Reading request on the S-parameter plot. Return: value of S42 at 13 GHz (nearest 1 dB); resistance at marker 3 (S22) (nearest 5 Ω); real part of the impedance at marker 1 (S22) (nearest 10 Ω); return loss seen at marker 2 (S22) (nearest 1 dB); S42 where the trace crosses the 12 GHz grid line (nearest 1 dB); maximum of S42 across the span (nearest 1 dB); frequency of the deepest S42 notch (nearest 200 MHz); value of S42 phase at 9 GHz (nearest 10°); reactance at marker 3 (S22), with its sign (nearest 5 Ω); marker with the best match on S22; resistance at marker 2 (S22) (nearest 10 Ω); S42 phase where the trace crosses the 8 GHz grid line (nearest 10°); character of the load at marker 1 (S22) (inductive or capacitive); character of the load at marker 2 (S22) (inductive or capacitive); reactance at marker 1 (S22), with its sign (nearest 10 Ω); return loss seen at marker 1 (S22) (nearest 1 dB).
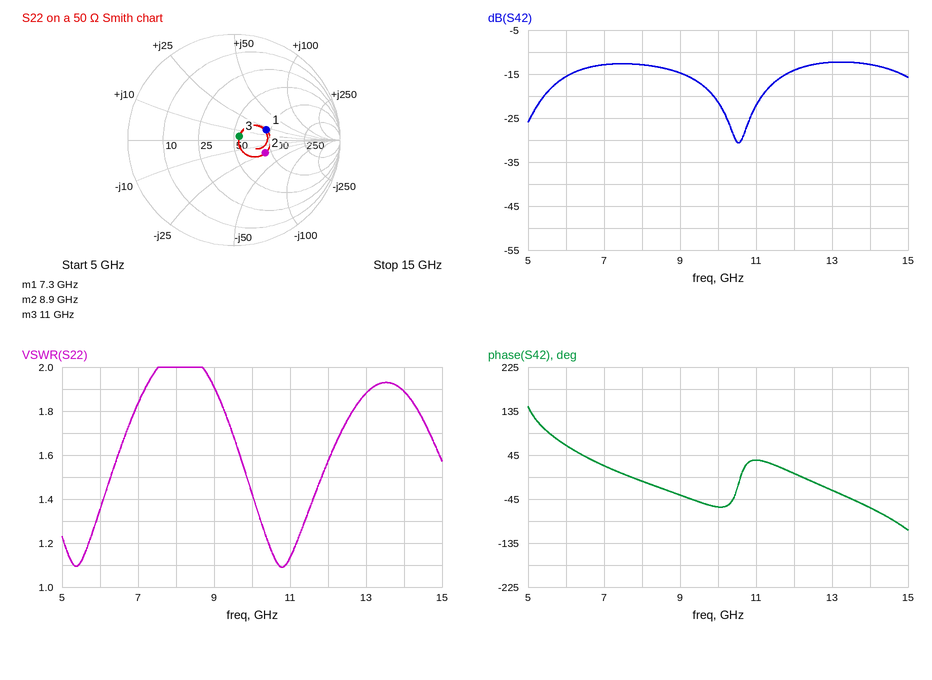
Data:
-12 dB
55 Ω
90 Ω
10 dB
-14 dB
-12 dB
10.6 GHz
-40°
+5 Ω
marker 3
90 Ω
-10°
inductive
capacitive
+20 Ω
10 dB
